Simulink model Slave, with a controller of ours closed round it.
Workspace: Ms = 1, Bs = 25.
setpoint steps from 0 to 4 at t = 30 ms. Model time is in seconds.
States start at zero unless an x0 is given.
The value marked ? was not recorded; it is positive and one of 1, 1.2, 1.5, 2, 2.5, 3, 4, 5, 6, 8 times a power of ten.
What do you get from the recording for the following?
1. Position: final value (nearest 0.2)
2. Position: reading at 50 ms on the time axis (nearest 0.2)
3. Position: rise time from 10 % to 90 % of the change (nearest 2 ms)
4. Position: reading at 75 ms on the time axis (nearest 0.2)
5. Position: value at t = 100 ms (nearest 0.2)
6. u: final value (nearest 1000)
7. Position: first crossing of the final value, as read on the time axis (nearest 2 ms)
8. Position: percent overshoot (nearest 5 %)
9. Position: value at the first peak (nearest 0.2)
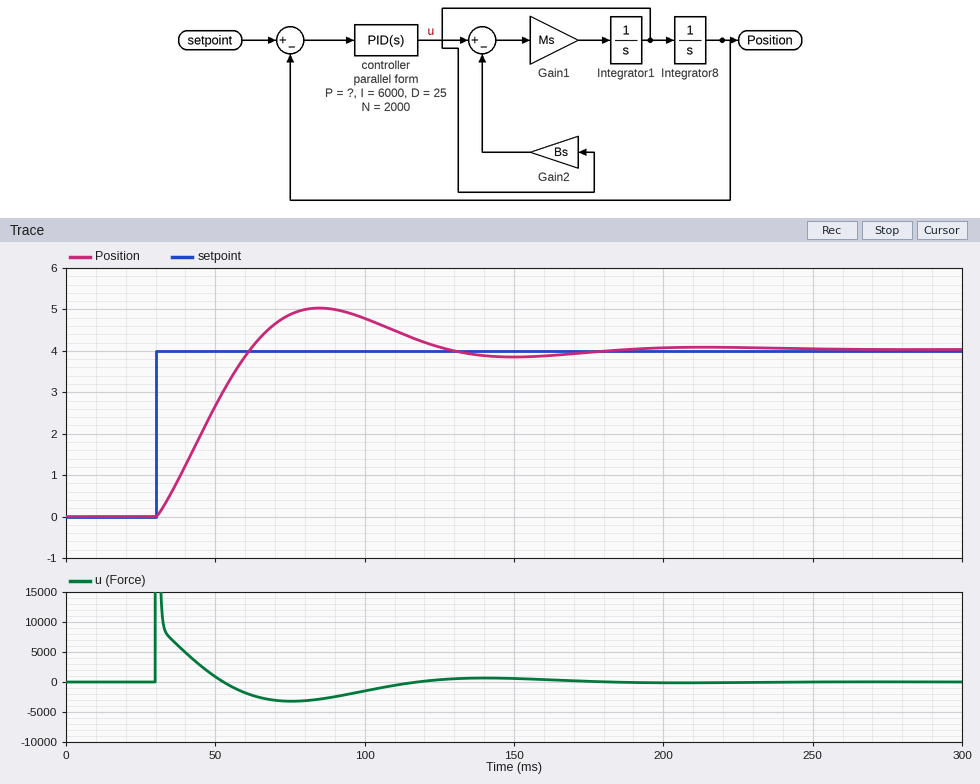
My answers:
4.0
2.6
24 ms
4.8
4.8
0
62 ms
25 %
5.0
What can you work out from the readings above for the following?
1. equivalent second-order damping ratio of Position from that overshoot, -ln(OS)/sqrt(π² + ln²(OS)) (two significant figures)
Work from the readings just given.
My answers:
0.40
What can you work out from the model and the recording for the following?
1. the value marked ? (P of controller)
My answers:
3000
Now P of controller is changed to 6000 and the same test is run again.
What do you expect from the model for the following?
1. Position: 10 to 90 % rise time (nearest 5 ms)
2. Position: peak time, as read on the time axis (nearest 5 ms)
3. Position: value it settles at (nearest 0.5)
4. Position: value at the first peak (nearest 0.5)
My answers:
15 ms
70 ms
4.0
5.5
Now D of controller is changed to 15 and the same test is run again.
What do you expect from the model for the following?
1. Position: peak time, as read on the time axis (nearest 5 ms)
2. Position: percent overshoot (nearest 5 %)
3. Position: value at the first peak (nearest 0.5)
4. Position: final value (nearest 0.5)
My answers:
85 ms
35 %
5.5
4.0
